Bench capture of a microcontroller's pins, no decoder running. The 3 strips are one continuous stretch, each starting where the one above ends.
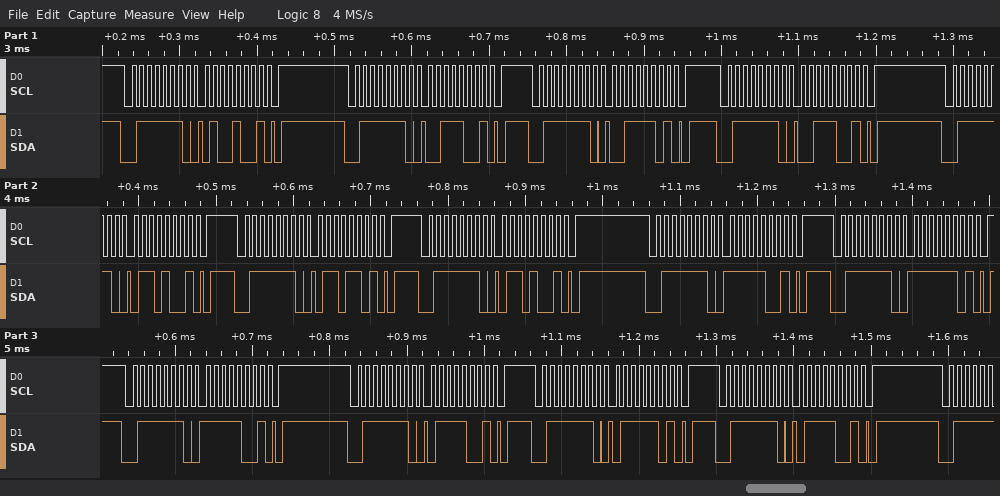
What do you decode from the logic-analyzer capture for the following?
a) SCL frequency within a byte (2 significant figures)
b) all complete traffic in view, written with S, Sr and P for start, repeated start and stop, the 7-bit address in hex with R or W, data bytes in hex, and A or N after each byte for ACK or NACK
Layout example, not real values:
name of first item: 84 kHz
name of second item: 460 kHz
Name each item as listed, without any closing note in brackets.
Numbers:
SCL frequency within a byte: 100 kHz
all complete traffic in view, written with S, Sr and P for start, repeated start and stop, the 7-bit address in hex with R or W, data bytes in hex, and A or N after each byte for ACK or NACK: S 3FW A 49 A P S 3FW A 39 A P S 3FW A 3D A P S 3FW A 39 A P S 3FW A 69 A P S 3FW A 6D A P S 3FW A 69 A P S 3FW A F9 A P S 3FW A FD A P S 3FW A F9 A P S 3FW A 79 A P S 3FW A 7D A P S 3FW A 79 A P
